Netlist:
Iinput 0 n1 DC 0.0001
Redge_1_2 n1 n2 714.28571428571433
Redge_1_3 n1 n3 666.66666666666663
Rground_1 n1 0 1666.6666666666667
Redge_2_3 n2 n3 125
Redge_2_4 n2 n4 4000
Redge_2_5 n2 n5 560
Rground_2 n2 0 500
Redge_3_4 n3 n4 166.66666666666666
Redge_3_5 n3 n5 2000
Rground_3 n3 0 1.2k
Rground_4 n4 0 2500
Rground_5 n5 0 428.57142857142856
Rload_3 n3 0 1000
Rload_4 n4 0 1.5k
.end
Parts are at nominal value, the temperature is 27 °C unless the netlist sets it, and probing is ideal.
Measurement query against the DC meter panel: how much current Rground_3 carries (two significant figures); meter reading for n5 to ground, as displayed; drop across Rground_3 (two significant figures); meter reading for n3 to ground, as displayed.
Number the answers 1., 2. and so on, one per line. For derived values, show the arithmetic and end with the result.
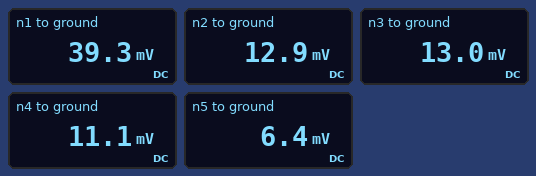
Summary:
1. (13 mV) / 1.2 kΩ = 11 µA
2. 6.4 mV
3. 13 mV = 13 mV
4. 13.0 mV
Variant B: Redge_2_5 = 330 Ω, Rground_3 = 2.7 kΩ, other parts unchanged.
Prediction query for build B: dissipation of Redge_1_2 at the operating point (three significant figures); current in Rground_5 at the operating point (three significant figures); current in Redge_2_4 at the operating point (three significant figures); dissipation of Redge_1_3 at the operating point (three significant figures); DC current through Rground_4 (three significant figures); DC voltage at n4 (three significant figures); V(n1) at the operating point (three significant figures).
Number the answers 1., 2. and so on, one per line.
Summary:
1. 990 nW
2. 18.6 µA
3. 349 nA
4. 1.01 µW
5. 4.69 µA
6. 11.7 mV
7. 39.7 mV
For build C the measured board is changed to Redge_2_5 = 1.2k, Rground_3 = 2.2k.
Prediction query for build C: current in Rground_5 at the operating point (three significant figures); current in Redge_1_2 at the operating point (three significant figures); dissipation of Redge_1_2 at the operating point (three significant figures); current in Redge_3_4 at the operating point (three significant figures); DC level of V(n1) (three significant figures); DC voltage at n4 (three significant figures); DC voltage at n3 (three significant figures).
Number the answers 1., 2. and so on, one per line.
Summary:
1. 12.3 µA
2. 36.6 µA
3. 955 nW
4. 12.7 µA
5. 40.6 mV
6. 12.4 mV
7. 14.5 mV
